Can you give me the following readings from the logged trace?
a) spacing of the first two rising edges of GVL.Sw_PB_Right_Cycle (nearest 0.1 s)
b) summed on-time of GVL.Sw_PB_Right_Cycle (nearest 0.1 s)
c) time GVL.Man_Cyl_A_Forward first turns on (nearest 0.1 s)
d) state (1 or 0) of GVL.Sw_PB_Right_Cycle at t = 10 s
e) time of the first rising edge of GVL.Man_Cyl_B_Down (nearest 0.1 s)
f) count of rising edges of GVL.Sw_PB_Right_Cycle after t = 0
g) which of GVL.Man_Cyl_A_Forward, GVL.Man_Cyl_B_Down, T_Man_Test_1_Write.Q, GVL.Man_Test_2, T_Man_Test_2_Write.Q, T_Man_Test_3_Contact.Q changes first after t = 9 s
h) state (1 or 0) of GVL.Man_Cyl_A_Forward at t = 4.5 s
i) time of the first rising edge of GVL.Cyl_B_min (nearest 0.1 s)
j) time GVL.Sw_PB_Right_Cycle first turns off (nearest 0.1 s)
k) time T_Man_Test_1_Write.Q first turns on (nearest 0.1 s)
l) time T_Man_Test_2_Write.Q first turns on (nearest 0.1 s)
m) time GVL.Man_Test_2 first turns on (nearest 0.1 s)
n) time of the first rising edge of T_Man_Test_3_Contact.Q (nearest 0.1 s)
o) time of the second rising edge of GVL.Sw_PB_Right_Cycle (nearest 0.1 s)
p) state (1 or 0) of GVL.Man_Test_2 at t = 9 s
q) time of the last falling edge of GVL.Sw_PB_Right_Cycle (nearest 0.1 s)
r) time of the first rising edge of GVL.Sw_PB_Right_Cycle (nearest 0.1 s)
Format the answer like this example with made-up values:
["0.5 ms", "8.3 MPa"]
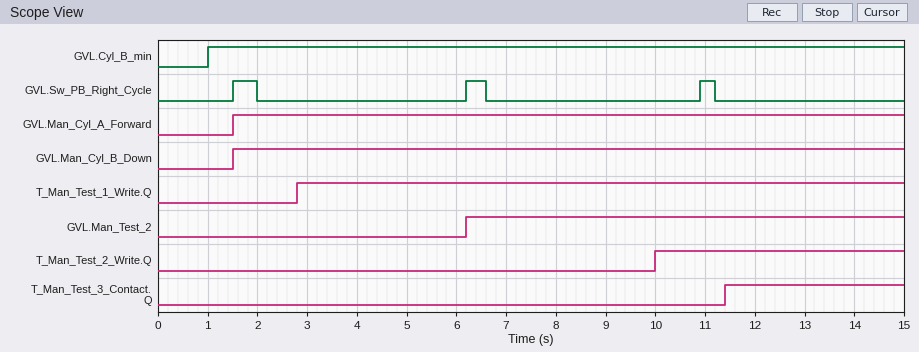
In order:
["4.7 s", "1.2 s", "1.5 s", "0", "1.5 s", "3", "T_Man_Test_2_Write.Q", "1", "1.0 s", "2.0 s", "2.8 s", "10.0 s", "6.2 s", "11.4 s", "6.2 s", "1", "11.2 s", "1.5 s"]
